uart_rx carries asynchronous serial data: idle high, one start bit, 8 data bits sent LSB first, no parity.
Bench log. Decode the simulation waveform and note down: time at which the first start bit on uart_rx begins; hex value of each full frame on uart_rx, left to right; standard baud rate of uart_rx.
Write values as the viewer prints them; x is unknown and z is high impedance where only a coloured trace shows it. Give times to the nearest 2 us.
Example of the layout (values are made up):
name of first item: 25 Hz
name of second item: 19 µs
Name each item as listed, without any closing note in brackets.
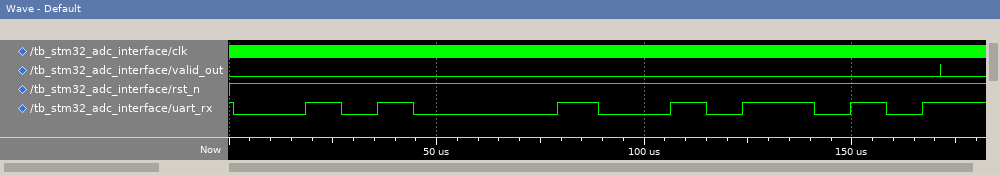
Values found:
time at which the first start bit on uart_rx begins: 0 us
hex value of each full frame on uart_rx, left to right: 0A, 5A
standard baud rate of uart_rx: 115200 baud
